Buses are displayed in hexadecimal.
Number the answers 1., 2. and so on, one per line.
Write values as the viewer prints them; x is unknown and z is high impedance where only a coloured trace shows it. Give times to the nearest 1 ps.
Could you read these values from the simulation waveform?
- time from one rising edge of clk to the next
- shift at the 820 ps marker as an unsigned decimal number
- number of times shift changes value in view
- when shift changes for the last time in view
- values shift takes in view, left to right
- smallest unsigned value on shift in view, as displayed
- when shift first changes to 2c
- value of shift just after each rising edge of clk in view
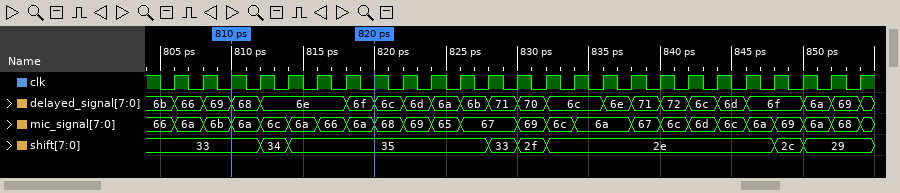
1. 2 ps
2. 53
3. 7
4. 850 ps
5. 33, 34, 35, 33, 2f, 2e, 2c, 29
6. 29
7. 848 ps
8. 33, 33, 33, 34, 35, 35, 35, 35, 35, 35, 35, 33, 2f, 2e, 2e, 2e, 2e, 2e, 2e, 2e, 2e, 2c, 29, 29, 29
